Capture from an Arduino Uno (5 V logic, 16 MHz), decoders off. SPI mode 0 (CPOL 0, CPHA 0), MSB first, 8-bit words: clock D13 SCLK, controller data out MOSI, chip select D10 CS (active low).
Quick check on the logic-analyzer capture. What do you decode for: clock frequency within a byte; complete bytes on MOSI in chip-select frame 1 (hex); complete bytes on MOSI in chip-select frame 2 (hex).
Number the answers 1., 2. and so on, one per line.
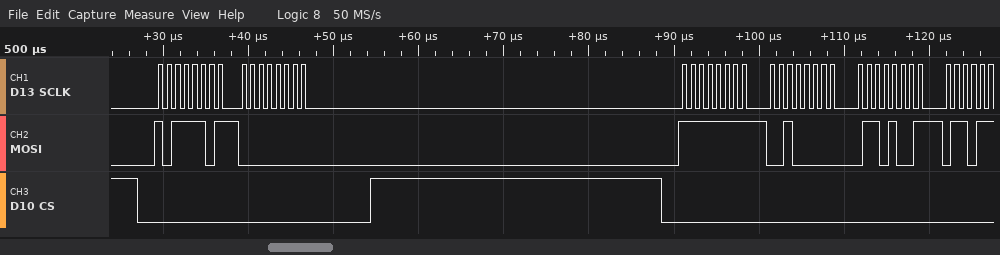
1. 1 MHz
2. 0xBD 0x00
3. 0xFF 0x20 0x69
